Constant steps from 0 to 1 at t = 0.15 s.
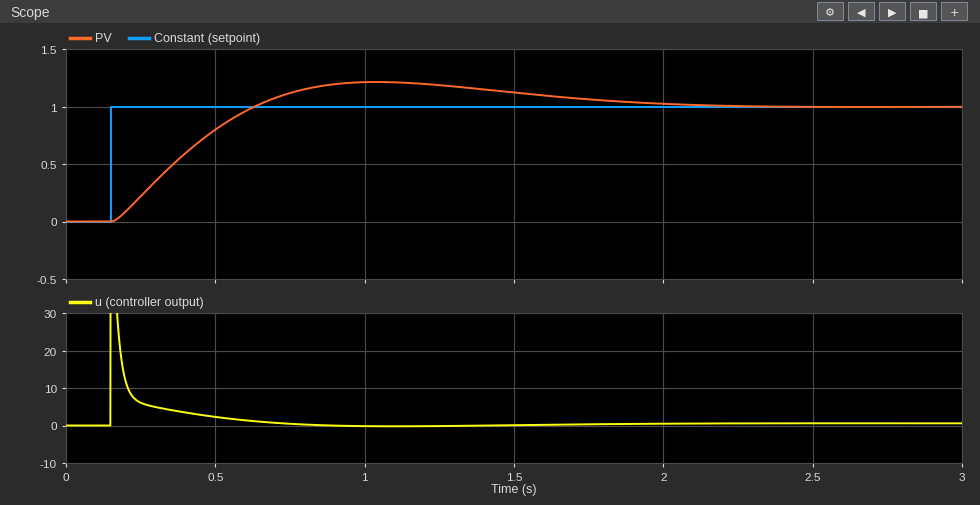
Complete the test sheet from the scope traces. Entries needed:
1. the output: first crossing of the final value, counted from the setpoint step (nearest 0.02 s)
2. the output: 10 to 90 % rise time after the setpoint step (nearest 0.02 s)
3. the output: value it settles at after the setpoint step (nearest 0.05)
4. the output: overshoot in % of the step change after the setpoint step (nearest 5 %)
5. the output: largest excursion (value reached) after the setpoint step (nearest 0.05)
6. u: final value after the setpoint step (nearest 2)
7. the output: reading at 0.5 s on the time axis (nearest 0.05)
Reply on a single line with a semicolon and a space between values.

0.48 s; 0.36 s; 1.00; 20 %; 1.20; 0; 0.80
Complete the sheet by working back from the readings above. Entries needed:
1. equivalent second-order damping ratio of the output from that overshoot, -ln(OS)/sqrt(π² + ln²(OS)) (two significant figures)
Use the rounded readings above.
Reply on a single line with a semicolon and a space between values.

0.46
